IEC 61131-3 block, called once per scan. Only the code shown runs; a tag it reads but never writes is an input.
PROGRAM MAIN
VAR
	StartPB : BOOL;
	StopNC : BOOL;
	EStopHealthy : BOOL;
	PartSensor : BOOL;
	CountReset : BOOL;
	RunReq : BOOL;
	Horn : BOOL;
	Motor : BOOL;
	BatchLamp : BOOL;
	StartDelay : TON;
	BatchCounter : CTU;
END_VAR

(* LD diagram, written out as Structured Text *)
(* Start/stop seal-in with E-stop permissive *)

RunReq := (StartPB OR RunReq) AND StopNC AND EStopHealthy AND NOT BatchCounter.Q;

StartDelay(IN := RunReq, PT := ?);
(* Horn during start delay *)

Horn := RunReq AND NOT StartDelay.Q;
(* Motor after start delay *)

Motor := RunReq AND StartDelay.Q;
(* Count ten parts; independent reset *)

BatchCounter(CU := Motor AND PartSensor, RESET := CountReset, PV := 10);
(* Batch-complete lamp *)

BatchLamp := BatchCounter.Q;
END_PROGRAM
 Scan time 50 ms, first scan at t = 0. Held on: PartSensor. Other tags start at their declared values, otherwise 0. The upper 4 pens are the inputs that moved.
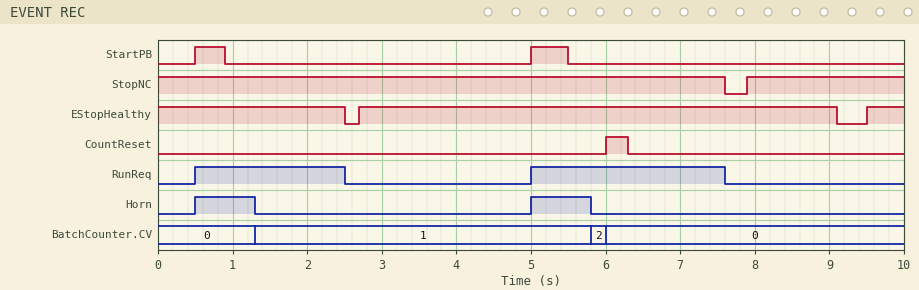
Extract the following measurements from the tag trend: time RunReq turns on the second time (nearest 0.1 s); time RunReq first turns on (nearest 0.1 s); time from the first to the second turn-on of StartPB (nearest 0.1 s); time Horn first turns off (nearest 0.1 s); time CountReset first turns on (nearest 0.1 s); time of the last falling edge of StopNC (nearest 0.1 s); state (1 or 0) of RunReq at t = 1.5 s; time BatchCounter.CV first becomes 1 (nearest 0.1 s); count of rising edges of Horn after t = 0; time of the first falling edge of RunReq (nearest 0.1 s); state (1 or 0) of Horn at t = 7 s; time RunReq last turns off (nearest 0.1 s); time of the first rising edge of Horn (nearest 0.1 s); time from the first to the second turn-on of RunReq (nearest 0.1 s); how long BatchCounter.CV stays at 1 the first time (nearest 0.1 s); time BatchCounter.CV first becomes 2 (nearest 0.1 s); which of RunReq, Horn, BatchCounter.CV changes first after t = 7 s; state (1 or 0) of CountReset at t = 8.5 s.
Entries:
5.0 s
0.5 s
4.5 s
1.3 s
6.0 s
7.6 s
1
1.3 s
2
2.5 s
0
7.6 s
0.5 s
4.5 s
4.5 s
5.8 s
RunReq
0
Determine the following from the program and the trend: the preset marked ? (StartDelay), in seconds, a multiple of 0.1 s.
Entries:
0.8 s
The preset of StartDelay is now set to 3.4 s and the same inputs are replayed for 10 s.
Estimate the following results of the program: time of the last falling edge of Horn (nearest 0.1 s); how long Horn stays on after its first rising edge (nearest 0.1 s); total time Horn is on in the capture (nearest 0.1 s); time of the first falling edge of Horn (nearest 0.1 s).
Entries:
7.6 s
2.0 s
4.6 s
2.5 s
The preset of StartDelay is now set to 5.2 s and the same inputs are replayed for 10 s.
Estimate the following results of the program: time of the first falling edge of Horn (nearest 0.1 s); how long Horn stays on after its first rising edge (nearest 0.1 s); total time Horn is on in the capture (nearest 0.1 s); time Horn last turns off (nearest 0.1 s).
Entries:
2.5 s
2.0 s
4.6 s
7.6 s
